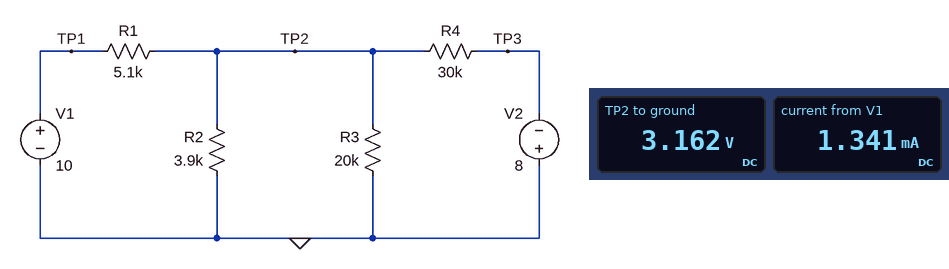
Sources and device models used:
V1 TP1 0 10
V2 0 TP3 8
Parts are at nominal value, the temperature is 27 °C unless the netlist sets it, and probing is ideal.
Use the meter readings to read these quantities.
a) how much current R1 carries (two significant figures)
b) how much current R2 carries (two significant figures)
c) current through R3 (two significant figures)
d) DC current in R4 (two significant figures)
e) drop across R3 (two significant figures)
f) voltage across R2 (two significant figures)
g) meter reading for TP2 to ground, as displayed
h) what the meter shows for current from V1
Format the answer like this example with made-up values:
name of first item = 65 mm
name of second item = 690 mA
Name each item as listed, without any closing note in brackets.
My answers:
how much current R1 carries = 1.3 mA
how much current R2 carries = 810 µA
current through R3 = 160 µA
DC current in R4 = 370 µA
drop across R3 = 3.2 V
voltage across R2 = 3.2 V
meter reading for TP2 to ground, as displayed = 3.162 V
what the meter shows for current from V1 = 1.341 mA
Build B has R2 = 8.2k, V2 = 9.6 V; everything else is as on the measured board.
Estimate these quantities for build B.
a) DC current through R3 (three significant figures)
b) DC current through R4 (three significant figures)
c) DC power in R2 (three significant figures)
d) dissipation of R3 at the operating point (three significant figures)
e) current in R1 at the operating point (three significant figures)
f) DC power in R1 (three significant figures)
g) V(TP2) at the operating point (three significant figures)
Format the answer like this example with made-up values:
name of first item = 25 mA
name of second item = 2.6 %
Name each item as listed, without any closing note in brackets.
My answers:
DC current through R3 = 204 µA
DC current through R4 = 456 µA
DC power in R2 = 2.04 mW
dissipation of R3 at the operating point = 836 µW
current in R1 at the operating point = 1.16 mA
DC power in R1 = 6.85 mW
V(TP2) at the operating point = 4.09 V
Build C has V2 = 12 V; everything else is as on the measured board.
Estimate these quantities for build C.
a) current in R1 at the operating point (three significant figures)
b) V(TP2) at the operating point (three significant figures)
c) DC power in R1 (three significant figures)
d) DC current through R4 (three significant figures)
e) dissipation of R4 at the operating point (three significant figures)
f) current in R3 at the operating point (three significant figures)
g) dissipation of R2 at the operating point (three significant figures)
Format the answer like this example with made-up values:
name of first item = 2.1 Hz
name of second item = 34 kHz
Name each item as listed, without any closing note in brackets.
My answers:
current in R1 at the operating point = 1.39 mA
V(TP2) at the operating point = 2.91 V
DC power in R1 = 9.85 mW
DC current through R4 = 497 µA
dissipation of R4 at the operating point = 7.41 mW
current in R3 at the operating point = 146 µA
dissipation of R2 at the operating point = 2.18 mW
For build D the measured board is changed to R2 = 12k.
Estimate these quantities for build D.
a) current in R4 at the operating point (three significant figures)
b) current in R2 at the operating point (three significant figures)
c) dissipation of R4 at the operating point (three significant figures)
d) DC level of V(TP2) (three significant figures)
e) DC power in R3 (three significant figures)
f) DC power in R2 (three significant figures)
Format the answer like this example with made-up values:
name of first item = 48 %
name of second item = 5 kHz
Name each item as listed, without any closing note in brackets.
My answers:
current in R4 at the operating point = 422 µA
current in R2 at the operating point = 389 µA
dissipation of R4 at the operating point = 5.35 mW
DC level of V(TP2) = 4.67 V
DC power in R3 = 1.09 mW
DC power in R2 = 1.82 mW
